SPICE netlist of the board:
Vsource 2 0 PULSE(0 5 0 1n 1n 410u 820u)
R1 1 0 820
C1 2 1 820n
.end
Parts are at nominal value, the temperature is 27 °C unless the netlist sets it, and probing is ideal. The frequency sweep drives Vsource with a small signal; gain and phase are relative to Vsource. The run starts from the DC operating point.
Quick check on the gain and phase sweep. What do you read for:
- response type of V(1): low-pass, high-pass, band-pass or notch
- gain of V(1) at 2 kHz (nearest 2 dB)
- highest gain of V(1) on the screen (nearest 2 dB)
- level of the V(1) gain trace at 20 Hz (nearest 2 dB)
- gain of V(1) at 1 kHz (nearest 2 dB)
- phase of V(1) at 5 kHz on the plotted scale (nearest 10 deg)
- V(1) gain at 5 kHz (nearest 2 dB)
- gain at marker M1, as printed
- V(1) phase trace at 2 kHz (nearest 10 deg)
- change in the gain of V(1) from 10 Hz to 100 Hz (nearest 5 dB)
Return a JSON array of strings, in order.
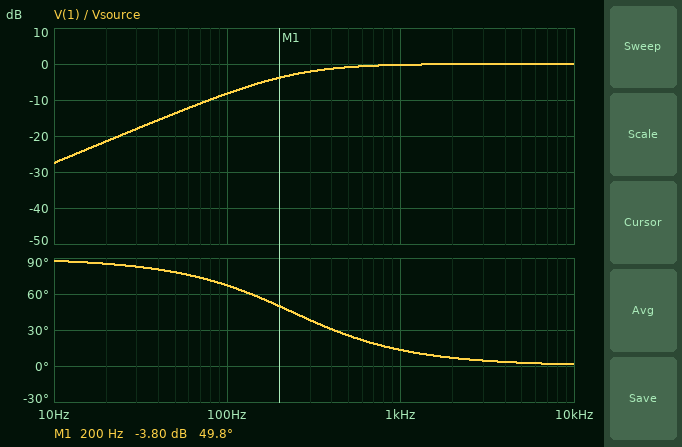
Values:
["high-pass", "0 dB", "0 dB", "-22 dB", "0 dB", "0 deg", "0 dB", "-3.80 dB", "10 deg", "20 dB"]
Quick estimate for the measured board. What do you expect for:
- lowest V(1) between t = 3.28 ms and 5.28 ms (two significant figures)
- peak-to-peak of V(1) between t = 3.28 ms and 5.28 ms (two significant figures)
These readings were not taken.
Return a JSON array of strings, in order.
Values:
["-3.2 V", "6.5 V"]
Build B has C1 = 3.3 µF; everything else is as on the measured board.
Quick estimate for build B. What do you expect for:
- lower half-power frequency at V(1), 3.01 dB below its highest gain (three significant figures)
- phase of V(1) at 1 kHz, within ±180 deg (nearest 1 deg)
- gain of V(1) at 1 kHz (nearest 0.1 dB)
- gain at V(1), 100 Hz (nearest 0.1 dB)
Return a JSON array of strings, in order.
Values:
["58.8 Hz", "3 deg", "0 dB", "-1.3 dB"]
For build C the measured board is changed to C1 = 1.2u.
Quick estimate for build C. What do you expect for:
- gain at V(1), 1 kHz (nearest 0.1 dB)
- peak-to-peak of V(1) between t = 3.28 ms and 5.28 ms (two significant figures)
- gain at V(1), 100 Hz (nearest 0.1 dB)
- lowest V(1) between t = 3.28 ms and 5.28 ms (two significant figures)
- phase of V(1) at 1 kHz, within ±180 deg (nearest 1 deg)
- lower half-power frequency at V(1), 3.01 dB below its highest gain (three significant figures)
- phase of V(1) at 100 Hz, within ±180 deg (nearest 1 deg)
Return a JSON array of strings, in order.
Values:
["-0.1 dB", "6.1 V", "-5.6 dB", "-3.0 V", "9 deg", "162 Hz", "58 deg"]
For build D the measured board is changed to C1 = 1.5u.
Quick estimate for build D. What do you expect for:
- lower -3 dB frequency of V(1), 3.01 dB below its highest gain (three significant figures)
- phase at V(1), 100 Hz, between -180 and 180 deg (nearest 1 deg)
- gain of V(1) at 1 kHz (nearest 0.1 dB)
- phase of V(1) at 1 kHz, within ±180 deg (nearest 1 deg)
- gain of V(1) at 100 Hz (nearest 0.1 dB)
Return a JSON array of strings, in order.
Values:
["129 Hz", "52 deg", "-0.1 dB", "7 deg", "-4.3 dB"]
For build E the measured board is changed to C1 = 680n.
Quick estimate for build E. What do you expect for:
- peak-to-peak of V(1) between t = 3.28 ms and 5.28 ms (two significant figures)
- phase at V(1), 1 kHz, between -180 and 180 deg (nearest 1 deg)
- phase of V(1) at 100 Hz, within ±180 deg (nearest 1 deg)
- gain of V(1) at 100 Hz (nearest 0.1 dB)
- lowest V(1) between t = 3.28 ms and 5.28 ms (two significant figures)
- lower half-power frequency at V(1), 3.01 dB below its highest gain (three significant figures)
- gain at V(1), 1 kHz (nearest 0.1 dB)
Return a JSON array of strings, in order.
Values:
["6.8 V", "16 deg", "71 deg", "-9.6 dB", "-3.4 V", "285 Hz", "-0.3 dB"]
